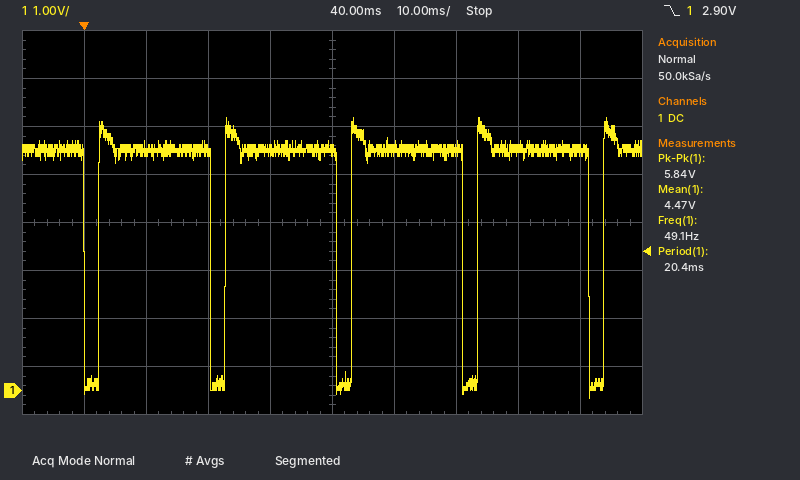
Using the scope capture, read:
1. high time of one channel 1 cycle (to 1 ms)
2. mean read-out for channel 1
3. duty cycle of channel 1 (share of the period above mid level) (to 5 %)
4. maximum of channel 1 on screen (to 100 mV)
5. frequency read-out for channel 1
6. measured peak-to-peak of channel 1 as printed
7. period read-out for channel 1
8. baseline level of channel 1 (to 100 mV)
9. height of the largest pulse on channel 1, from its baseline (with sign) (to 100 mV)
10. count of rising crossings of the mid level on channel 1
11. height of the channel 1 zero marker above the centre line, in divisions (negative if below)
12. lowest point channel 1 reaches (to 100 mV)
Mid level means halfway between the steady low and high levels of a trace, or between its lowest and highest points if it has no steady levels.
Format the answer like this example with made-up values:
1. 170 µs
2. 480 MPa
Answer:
1. 18 ms
2. 4.47 V
3. 90 %
4. 5.7 V
5. 49.1 Hz
6. 5.84 V
7. 20.4 ms
8. 5.0 V
9. -5.2 V
10. 5
11. -3.5 div
12. -200 mV
